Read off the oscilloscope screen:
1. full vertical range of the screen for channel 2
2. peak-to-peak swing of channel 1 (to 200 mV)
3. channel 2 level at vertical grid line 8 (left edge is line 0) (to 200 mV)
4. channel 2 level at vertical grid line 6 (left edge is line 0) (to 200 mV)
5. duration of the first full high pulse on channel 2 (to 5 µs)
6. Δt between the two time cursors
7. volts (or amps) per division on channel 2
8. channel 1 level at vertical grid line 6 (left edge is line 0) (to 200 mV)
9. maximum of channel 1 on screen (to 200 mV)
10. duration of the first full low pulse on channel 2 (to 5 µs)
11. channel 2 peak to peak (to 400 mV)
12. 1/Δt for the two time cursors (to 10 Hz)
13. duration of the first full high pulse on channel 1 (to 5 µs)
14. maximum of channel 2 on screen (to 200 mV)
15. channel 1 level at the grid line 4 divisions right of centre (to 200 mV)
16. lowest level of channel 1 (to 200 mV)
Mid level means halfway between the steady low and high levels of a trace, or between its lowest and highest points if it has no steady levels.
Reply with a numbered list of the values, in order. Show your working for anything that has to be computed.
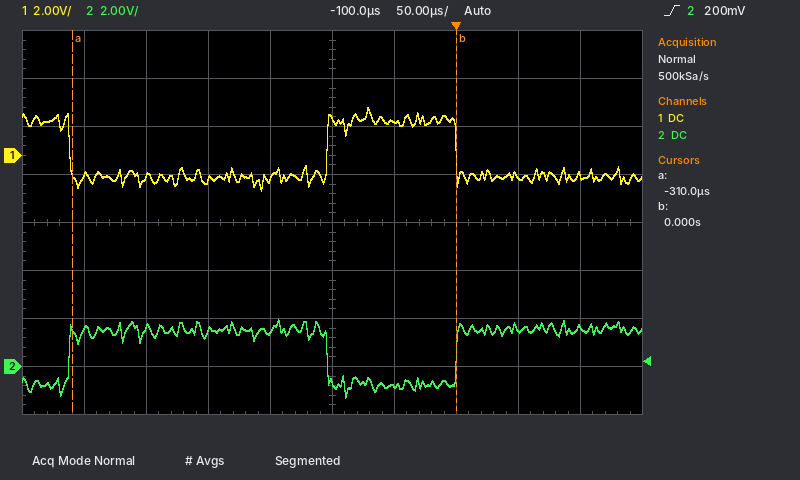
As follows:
1. 16 V
2. 2.0 V − (-1.4 V) = 3.4 V
3. 1.6 V
4. -800 mV
5. 210 µs
6. 0 s − (-310 µs) = 310 µs
7. 2 V
8. 1.4 V
9. 2.0 V
10. 105 µs
11. 3.2 V
12. 1 / 310 µs ≈ 3.23 kHz
13. 105 µs
14. 2.0 V
15. -800 mV
16. -1.4 V
